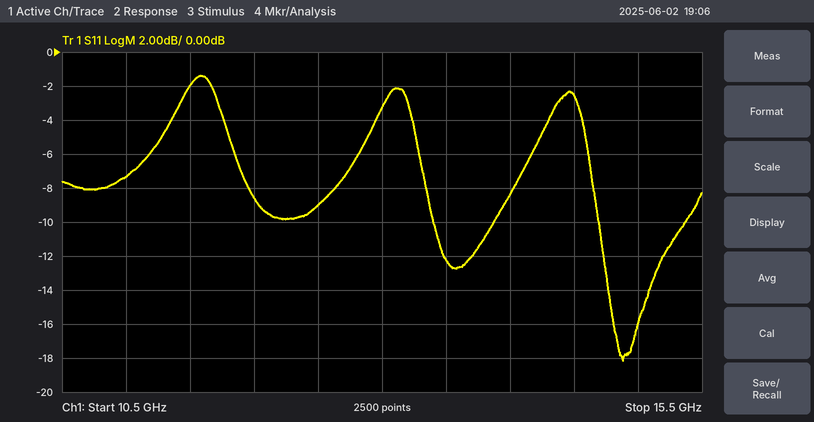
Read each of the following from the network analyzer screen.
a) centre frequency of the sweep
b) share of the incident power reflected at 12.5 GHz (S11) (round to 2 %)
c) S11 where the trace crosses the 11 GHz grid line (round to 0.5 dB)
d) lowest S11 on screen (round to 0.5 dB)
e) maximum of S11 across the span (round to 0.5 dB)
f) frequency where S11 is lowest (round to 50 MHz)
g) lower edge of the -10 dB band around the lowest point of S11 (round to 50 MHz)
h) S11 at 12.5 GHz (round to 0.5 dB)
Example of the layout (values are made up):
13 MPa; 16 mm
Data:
13 GHz; 12 %; -7.5 dB; -18.0 dB; -1.5 dB; 14.90 GHz; 14.70 GHz; -9.0 dB
